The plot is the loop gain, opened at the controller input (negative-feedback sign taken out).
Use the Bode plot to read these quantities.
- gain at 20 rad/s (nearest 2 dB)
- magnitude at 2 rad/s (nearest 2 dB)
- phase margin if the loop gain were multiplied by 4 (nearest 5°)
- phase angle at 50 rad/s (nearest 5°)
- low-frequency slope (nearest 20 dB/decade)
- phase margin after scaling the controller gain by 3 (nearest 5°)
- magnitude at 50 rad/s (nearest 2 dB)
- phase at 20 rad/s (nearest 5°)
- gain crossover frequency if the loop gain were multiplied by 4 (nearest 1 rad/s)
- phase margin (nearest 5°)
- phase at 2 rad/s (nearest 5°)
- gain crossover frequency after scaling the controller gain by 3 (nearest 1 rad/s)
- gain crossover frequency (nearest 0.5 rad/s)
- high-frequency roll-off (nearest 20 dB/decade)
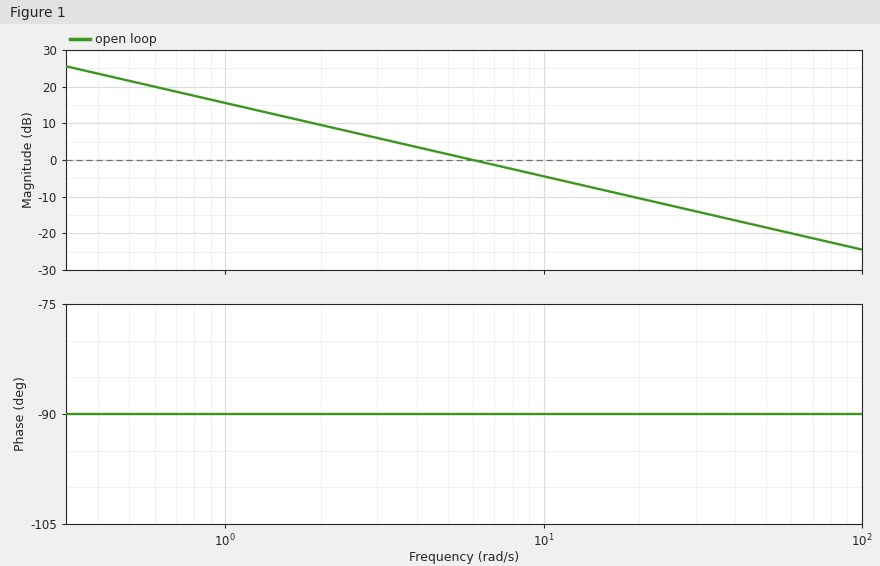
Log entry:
-10 dB
10 dB
90°
-90°
-20 dB/decade
90°
-18 dB
-90°
24 rad/s
90°
-90°
18 rad/s
6.0 rad/s
-20 dB/decade
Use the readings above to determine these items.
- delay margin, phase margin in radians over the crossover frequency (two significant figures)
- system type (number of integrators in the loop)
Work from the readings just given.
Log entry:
0.26 s
1
